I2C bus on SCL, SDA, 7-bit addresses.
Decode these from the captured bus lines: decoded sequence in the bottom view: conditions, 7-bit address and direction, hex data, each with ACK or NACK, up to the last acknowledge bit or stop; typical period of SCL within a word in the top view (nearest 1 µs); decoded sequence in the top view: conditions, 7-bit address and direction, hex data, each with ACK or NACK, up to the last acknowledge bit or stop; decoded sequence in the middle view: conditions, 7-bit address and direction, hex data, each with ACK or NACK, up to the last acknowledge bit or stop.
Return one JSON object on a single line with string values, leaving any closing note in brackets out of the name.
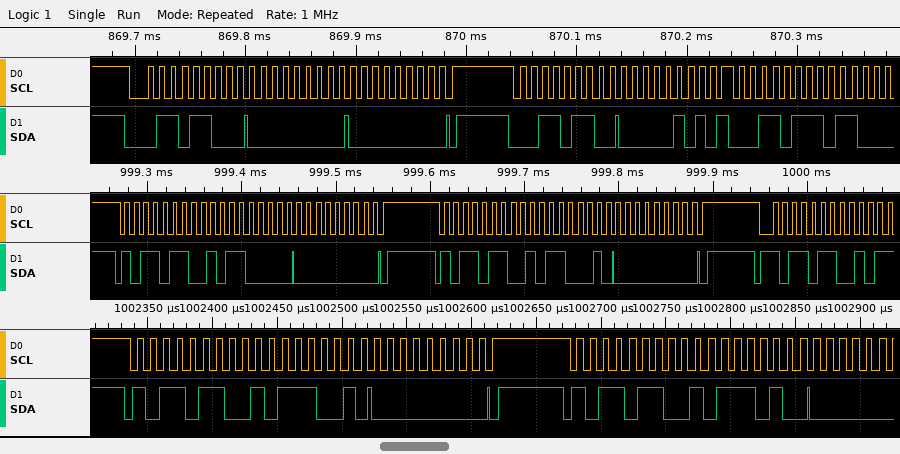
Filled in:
{"decoded sequence in the bottom view: conditions, 7-bit address and direction, hex data, each with ACK or NACK, up to the last acknowledge bit or stop": "start, address 5B write ACK, B9 ACK, 00 ACK, stop, start, address 5B write ACK, BA ACK", "typical period of SCL within a word in the top view": "10 µs", "decoded sequence in the top view: conditions, 7-bit address and direction, hex data, each with ACK or NACK, up to the last acknowledge bit or stop": "start, address 36 write ACK, 00 ACK, 00 ACK, stop, start, address 1B write ACK, 05 ACK, repeated start, address 1B read ACK", "decoded sequence in the middle view: conditions, 7-bit address and direction, hex data, each with ACK or NACK, up to the last acknowledge bit or stop": "start, address 5B write ACK, B0 ACK, 00 ACK, stop, start, address 5B write ACK, B1 ACK, 00 ACK, stop, start, address 5B write ACK"}
